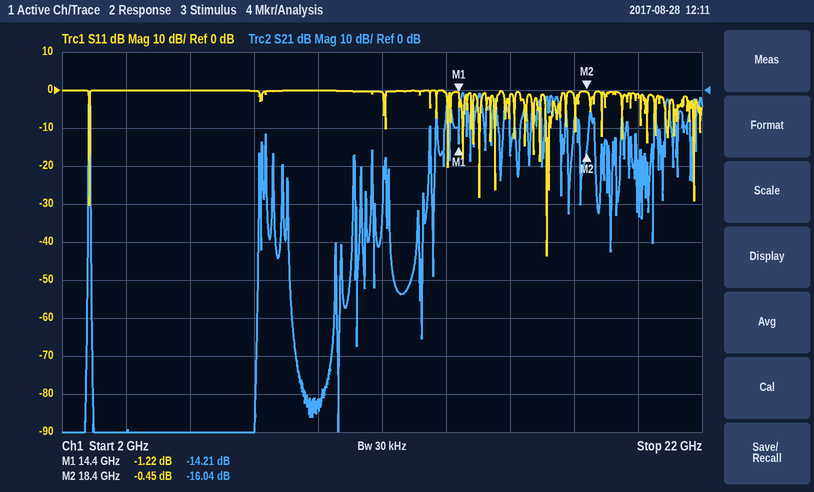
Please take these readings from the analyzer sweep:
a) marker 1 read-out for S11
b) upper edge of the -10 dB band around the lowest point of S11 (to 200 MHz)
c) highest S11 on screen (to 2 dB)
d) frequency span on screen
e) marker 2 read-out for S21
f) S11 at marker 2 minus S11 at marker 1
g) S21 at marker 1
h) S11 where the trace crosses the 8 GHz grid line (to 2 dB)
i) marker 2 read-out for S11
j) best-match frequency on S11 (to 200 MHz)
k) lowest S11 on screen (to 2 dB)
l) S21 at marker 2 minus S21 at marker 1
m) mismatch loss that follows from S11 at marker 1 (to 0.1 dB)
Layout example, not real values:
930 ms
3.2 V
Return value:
-1.22 dB
17.2 GHz
0 dB
20 GHz
-16.04 dB
0.77 dB
-14.21 dB
0 dB
-0.45 dB
17.2 GHz
-44 dB
-1.83 dB
6.1 dB
